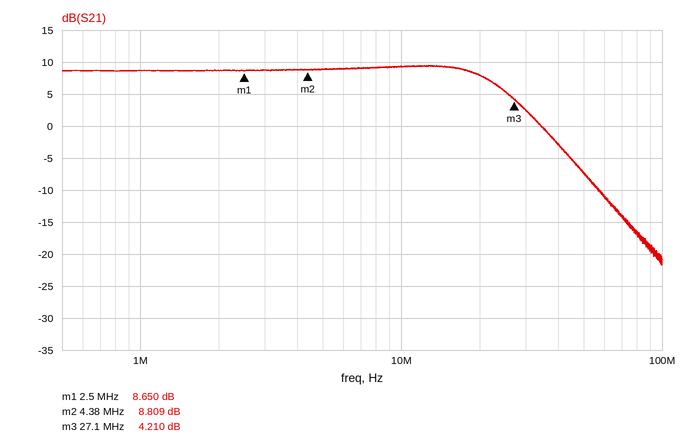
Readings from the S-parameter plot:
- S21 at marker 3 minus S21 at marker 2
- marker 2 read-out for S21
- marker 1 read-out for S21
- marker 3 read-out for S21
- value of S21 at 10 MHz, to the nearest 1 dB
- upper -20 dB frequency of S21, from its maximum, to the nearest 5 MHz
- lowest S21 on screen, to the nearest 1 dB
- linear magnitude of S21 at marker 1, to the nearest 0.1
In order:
-4.599 dB
8.809 dB
8.650 dB
4.210 dB
9 dB
60 MHz
-22 dB
2.7
